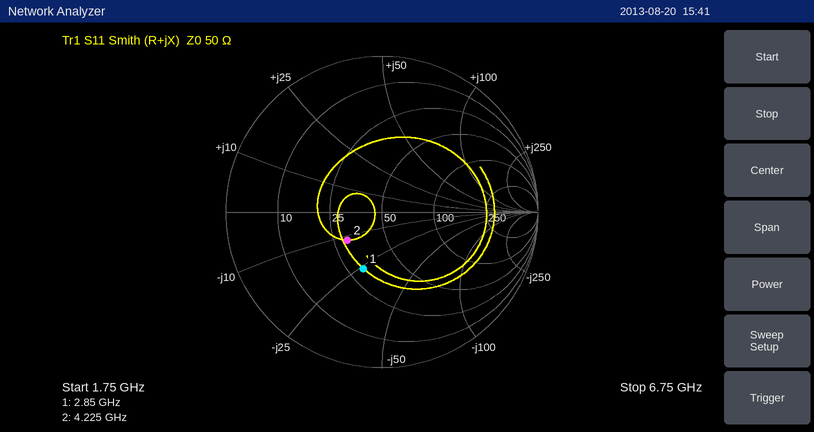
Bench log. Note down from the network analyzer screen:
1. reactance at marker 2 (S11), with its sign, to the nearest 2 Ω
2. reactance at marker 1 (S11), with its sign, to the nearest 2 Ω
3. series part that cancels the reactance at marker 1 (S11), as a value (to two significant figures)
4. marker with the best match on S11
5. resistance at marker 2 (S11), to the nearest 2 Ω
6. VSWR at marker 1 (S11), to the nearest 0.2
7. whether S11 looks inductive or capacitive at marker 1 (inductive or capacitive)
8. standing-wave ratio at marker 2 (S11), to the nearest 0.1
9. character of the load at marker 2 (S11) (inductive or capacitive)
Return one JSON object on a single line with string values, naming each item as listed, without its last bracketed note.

{"reactance at marker 2 (S11), with its sign, to the nearest 2 Ω": "-12 Ω", "reactance at marker 1 (S11), with its sign, to the nearest 2 Ω": "-26 Ω", "series part that cancels the reactance at marker 1 (S11), as a value": "1.5 nH", "marker with the best match on S11": "marker 2", "resistance at marker 2 (S11), to the nearest 2 Ω": "30 Ω", "VSWR at marker 1 (S11), to the nearest 0.2": "2.2", "whether S11 looks inductive or capacitive at marker 1": "capacitive", "standing-wave ratio at marker 2 (S11), to the nearest 0.1": "1.8", "character of the load at marker 2 (S11)": "capacitive"}
